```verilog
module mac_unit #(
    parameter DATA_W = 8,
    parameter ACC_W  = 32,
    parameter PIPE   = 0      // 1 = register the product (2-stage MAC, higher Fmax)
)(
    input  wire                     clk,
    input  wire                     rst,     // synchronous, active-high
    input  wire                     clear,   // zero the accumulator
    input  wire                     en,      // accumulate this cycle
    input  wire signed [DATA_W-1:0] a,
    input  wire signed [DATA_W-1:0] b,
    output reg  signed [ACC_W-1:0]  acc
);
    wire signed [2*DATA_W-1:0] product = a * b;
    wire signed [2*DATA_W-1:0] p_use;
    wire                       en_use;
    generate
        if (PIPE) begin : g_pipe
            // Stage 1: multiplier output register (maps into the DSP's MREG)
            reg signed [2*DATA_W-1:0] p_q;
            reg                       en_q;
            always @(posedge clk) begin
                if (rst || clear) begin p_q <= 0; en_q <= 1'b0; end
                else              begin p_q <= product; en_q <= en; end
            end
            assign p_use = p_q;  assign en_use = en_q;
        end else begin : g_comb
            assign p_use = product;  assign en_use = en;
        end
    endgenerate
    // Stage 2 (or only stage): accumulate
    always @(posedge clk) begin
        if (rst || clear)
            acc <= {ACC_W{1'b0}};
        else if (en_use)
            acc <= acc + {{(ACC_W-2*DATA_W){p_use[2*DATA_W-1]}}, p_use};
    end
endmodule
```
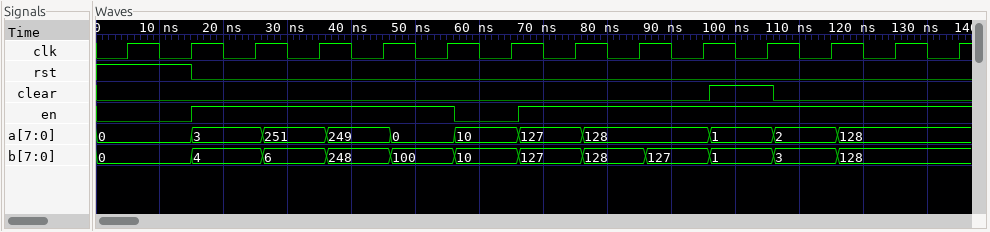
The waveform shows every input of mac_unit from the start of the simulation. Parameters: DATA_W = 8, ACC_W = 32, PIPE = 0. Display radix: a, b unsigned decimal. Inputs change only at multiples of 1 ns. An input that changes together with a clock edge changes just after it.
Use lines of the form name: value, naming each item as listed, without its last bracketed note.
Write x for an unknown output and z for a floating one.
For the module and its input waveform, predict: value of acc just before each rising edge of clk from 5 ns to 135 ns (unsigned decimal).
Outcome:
value of acc just before each rising edge of clk from 5 ns to 135 ns: x, 0, 0, 12, 4294967278, 38, 38, 38, 16167, 32551, 16295, 0, 6, 16390
